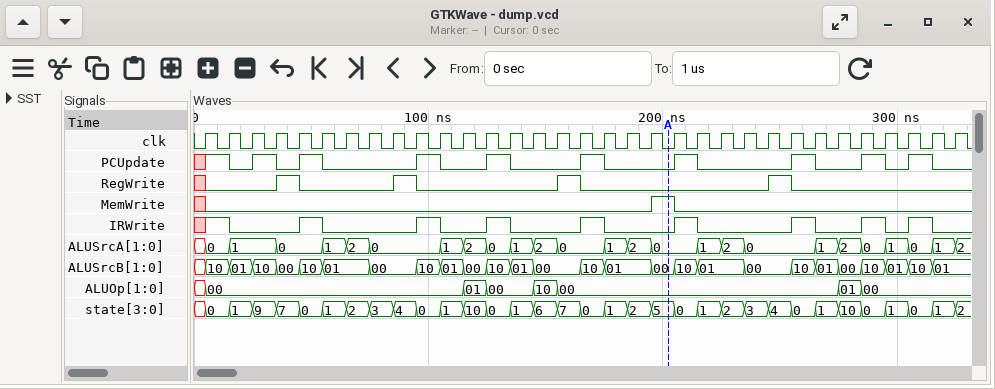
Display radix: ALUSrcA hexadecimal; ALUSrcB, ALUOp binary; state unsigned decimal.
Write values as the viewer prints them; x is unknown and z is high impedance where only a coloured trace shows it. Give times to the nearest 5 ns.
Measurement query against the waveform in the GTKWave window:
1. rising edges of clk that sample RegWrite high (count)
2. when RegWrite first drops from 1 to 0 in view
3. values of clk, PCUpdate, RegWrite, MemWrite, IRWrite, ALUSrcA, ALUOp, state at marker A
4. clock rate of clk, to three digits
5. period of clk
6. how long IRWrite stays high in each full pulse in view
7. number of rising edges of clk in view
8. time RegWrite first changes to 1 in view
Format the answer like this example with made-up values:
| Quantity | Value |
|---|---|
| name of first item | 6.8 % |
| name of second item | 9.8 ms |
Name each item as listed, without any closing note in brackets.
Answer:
| Quantity | Value |
|---|---|
| rising edges of clk that sample RegWrite high | 4 |
| when RegWrite first drops from 1 to 0 in view | 45 ns |
| values of clk, PCUpdate, RegWrite, MemWrite, IRWrite, ALUSrcA, ALUOp, state at marker A | clk=0, PCUpdate=0, RegWrite=0, MemWrite=1, IRWrite=0, ALUSrcA=0, ALUOp=00, state=5 |
| clock rate of clk, to three digits | 100 MHz |
| period of clk | 10 ns |
| how long IRWrite stays high in each full pulse in view | 10 ns, 10 ns, 10 ns, 10 ns, 10 ns, 10 ns, 10 ns, 10 ns |
| number of rising edges of clk in view | 33 |
| time RegWrite first changes to 1 in view | 35 ns |
